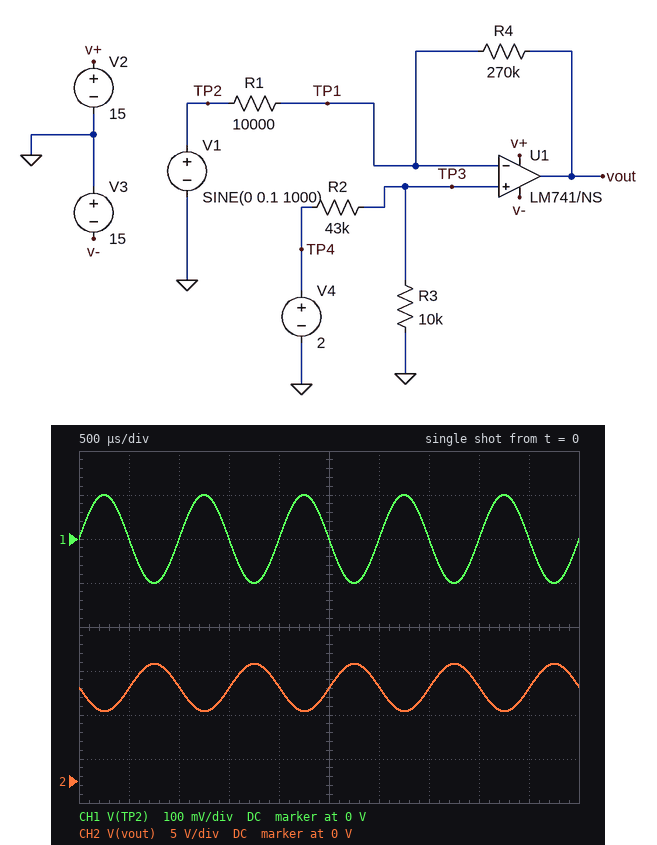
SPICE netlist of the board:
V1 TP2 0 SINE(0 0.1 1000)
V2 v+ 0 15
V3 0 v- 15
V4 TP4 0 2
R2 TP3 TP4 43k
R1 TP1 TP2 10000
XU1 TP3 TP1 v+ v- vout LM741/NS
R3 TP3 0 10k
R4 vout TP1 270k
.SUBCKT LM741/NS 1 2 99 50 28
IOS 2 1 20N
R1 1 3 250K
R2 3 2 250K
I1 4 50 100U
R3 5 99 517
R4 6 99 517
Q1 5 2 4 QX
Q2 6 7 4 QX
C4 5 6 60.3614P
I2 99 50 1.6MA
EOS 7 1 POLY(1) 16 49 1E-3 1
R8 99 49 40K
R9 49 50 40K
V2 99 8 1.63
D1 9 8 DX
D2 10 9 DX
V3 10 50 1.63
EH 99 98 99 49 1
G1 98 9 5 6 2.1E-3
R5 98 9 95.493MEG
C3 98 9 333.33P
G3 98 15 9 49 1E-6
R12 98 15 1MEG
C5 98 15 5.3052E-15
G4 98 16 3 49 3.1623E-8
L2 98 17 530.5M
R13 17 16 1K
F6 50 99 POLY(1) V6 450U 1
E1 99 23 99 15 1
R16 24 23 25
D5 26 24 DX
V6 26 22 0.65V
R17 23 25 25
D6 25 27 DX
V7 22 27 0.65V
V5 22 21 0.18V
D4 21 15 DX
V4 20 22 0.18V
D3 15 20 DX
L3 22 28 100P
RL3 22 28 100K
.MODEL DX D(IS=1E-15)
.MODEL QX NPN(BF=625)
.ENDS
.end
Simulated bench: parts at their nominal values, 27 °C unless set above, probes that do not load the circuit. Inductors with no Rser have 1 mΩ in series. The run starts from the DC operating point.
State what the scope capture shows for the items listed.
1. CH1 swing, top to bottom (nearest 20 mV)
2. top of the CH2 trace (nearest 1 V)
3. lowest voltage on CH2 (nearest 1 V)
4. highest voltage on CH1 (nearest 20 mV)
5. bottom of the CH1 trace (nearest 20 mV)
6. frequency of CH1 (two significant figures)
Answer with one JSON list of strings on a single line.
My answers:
["200 mV", "13 V", "8 V", "100 mV", "-100 mV", "1.0 kHz"]
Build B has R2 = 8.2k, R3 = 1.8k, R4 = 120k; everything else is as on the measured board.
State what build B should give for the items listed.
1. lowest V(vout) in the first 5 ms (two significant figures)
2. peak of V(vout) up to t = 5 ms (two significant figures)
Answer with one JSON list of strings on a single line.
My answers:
["3.5 V", "5.9 V"]
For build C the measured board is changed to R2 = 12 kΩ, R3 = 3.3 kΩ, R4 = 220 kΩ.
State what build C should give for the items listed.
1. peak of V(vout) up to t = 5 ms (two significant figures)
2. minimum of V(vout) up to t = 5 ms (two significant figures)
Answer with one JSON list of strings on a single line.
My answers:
["12 V", "7.8 V"]
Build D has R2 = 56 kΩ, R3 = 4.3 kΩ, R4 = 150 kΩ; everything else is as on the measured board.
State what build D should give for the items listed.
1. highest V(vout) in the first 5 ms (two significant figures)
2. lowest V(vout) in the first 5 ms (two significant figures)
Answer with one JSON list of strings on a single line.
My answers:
["3.8 V", "810 mV"]
